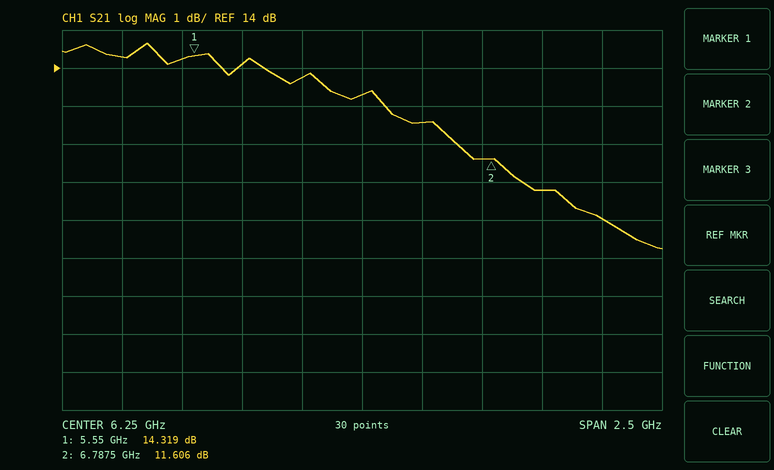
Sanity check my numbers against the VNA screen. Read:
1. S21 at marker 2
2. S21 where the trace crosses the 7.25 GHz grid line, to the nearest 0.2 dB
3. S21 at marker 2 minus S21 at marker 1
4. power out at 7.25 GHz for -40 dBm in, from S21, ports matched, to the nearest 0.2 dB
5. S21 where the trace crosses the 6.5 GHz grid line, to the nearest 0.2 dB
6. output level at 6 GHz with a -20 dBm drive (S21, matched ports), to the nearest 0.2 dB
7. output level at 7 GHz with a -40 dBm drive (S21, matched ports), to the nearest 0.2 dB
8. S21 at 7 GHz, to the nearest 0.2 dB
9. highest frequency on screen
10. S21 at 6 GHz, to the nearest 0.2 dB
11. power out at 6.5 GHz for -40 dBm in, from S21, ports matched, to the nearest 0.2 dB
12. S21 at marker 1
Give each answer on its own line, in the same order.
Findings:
11.606 dB
10.0 dB
-2.713 dB
-30.0 dBm
12.6 dB
-6.2 dBm
-29.2 dBm
10.8 dB
7.5 GHz
13.8 dB
-27.4 dBm
14.319 dB
